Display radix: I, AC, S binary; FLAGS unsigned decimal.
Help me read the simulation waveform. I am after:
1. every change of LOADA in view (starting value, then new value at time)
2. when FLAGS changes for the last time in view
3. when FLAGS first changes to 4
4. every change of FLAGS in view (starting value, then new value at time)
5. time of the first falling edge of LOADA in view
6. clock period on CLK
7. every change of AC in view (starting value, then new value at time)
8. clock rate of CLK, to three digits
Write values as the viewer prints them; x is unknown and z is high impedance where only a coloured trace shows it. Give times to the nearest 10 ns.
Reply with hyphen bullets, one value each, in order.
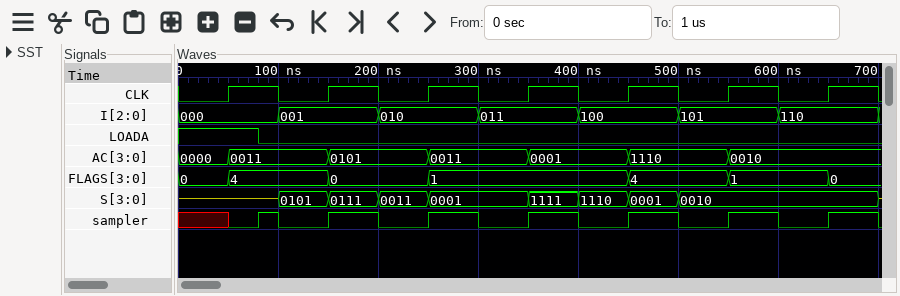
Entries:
- 1, 0 at 80 ns
- 650 ns
- 50 ns
- 0, 4 at 50 ns, 0 at 150 ns, 1 at 250 ns, 4 at 450 ns, 1 at 550 ns, 0 at 650 ns
- 80 ns
- 100 ns
- 0000, 0011 at 50 ns, 0101 at 150 ns, 0011 at 250 ns, 0001 at 350 ns, 1110 at 450 ns, 0010 at 550 ns
- 10.0 MHz
